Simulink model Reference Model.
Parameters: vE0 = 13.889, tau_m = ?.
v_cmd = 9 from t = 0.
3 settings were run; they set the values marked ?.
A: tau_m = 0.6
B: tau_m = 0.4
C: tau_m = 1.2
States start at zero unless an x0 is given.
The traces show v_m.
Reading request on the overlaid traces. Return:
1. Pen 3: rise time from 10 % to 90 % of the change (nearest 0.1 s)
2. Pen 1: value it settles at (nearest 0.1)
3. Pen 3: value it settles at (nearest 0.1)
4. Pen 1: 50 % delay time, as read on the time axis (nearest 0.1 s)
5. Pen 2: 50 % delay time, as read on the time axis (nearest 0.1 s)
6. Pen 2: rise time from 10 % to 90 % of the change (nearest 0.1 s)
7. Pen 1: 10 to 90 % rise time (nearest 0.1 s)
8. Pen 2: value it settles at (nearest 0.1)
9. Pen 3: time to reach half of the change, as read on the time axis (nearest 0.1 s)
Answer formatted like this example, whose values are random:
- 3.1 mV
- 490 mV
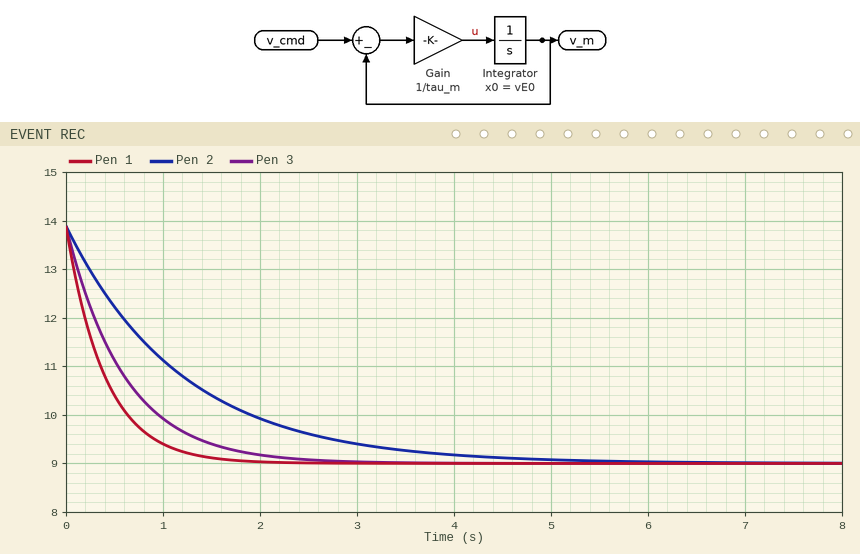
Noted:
- 1.3 s
- 9.0
- 9.0
- 0.3 s
- 0.8 s
- 2.6 s
- 0.9 s
- 9.0
- 0.4 s
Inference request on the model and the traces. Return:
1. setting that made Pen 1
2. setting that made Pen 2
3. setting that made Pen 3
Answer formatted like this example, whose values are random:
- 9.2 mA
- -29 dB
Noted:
- B
- C
- A
